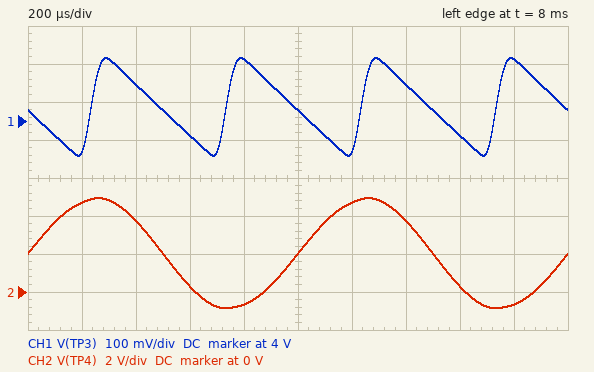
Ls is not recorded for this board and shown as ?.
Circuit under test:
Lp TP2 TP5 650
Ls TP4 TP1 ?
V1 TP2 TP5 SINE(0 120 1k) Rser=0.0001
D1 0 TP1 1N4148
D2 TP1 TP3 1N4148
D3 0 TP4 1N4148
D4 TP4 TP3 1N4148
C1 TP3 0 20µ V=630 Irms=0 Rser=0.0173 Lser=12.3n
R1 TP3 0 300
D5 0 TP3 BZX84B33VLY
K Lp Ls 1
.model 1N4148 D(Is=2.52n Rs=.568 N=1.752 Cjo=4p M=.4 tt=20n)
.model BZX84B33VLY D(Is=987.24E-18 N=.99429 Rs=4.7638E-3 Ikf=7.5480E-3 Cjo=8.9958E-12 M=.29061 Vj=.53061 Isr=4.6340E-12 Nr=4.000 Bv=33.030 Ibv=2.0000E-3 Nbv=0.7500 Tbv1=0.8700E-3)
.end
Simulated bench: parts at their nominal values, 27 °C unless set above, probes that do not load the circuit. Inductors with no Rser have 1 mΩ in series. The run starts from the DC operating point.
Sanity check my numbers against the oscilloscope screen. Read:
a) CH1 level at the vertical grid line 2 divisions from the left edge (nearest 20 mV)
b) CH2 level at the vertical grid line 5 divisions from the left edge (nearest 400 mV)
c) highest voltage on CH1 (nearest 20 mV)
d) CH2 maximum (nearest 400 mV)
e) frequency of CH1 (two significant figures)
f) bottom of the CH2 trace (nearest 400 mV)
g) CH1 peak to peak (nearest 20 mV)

4.10 V
2.0 V
4.16 V
4.8 V
2.0 kHz
-800 mV
260 mV
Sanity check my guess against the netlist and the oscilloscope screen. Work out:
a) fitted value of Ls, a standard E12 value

1.5 H
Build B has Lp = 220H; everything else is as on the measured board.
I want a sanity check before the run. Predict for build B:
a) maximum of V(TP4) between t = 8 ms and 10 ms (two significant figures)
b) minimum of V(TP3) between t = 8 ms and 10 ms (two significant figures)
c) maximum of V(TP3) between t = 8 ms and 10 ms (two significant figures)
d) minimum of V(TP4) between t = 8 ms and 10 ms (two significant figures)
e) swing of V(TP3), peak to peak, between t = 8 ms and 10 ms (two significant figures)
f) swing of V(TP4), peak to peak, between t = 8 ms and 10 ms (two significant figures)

9.0 V
7.7 V
8.2 V
-950 mV
520 mV
10 V
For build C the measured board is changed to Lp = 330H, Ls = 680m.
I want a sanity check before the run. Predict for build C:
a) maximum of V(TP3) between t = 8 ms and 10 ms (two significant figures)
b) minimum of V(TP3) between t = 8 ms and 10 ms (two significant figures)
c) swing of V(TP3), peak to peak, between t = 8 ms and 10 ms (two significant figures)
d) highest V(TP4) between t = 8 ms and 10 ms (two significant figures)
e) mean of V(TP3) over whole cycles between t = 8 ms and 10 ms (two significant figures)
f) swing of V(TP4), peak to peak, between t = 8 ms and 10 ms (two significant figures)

3.9 V
3.6 V
240 mV
4.6 V
3.7 V
5.5 V
